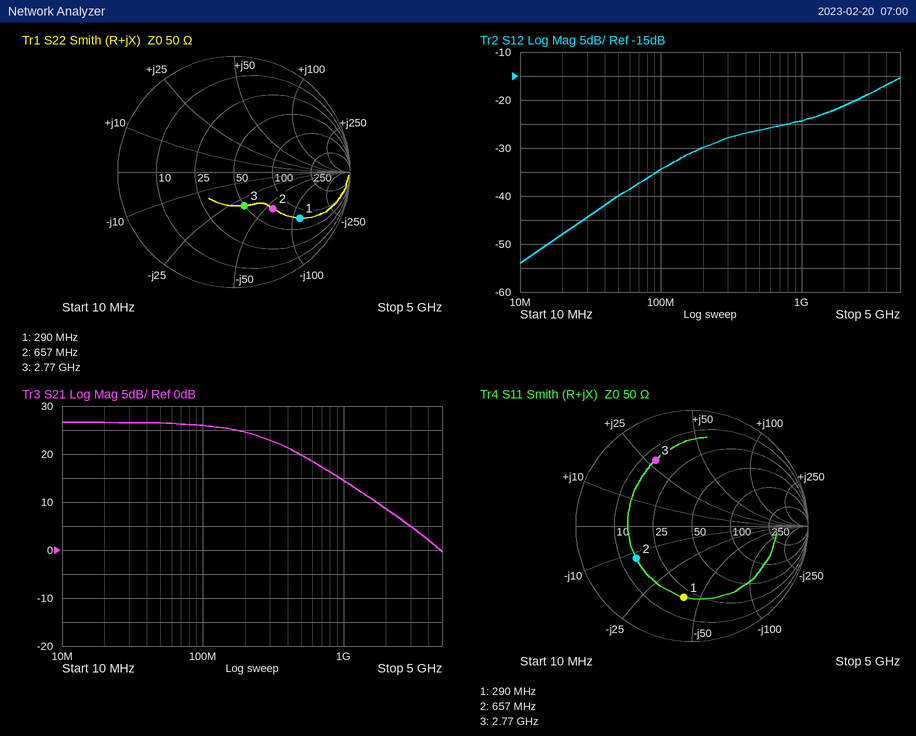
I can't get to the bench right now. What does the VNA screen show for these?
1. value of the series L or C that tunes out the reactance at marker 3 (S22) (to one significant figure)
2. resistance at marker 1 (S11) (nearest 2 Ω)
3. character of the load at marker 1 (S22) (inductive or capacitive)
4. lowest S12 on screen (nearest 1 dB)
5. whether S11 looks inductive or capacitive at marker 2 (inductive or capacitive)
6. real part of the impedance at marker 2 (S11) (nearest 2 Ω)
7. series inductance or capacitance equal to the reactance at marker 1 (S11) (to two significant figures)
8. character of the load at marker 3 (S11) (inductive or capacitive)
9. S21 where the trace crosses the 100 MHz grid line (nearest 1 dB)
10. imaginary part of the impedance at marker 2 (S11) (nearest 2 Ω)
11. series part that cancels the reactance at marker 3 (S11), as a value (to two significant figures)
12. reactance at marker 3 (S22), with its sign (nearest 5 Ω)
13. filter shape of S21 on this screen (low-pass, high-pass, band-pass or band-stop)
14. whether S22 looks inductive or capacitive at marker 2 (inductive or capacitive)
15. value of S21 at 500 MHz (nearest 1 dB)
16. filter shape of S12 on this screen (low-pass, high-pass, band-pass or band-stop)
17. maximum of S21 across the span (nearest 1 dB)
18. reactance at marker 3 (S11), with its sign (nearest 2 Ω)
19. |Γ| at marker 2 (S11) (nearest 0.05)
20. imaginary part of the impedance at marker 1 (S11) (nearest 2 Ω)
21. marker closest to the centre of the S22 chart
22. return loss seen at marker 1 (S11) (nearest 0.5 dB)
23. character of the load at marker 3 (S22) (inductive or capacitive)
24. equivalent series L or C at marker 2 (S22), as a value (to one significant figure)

2 nH
20 Ω
capacitive
-54 dB
capacitive
16 Ω
14 pF
inductive
26 dB
-12 Ω
2.1 pF
-30 Ω
low-pass
capacitive
20 dB
high-pass
27 dB
+28 Ω
0.55
-40 Ω
marker 3
4.0 dB
capacitive
4 pF
